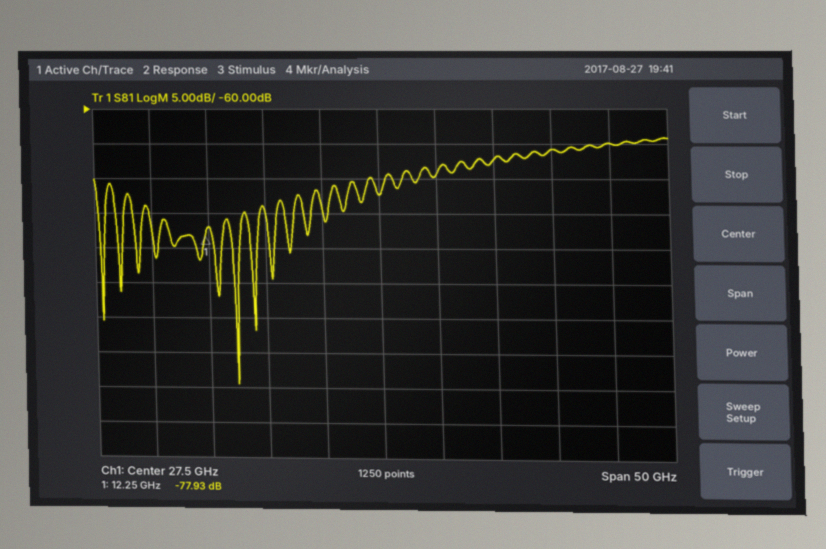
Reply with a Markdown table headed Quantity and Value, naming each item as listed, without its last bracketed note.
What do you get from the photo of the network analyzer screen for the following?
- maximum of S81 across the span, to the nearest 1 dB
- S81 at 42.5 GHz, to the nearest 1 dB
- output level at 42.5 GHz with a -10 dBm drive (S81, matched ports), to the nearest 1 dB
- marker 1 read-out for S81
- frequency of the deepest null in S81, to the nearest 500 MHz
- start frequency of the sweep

| Quantity | Value |
|---|---|
| maximum of S81 across the span, to the nearest 1 dB | -64 dB |
| S81 at 42.5 GHz, to the nearest 1 dB | -66 dB |
| output level at 42.5 GHz with a -10 dBm drive (S81, matched ports), to the nearest 1 dB | -76 dBm |
| marker 1 read-out for S81 | -77.93 dB |
| frequency of the deepest null in S81, to the nearest 500 MHz | 15.0 GHz |
| start frequency of the sweep | 2.5 GHz |
